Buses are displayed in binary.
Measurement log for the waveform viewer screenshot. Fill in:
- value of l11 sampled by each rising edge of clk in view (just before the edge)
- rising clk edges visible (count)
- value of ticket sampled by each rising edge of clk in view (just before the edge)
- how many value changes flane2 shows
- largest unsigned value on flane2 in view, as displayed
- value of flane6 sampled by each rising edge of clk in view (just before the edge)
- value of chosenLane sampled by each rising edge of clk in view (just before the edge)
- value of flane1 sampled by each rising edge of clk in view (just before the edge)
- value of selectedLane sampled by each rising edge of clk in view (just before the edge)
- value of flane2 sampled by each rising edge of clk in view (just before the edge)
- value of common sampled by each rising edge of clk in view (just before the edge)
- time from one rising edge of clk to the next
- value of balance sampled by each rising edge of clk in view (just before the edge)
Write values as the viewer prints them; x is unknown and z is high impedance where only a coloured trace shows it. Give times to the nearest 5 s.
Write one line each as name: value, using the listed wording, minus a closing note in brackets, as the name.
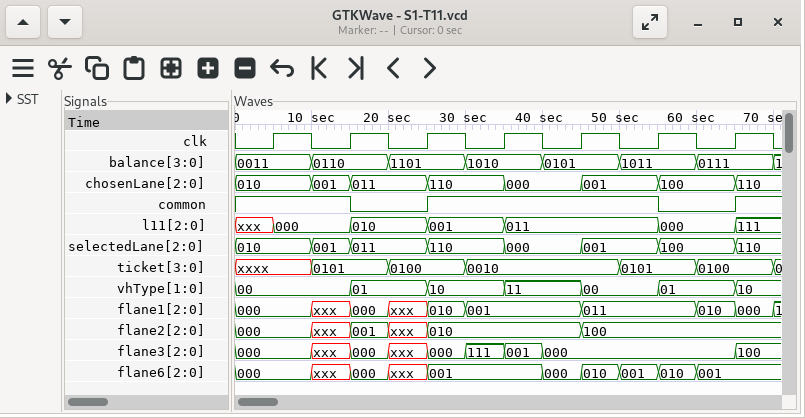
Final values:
value of l11 sampled by each rising edge of clk in view: xxx, 000, 010, 001, 011, 011, 000
rising clk edges visible: 7
value of ticket sampled by each rising edge of clk in view: xxxx, 0101, 0100, 0010, 0010, 0101, 0100
how many value changes flane2 shows: 5
largest unsigned value on flane2 in view, as displayed: 100
value of flane6 sampled by each rising edge of clk in view: 000, xxx, xxx, 001, 000, 001, 001
value of chosenLane sampled by each rising edge of clk in view: 010, 001, 011, 110, 000, 001, 100
value of flane1 sampled by each rising edge of clk in view: 000, xxx, xxx, 001, 001, 011, 010
value of selectedLane sampled by each rising edge of clk in view: 010, 001, 011, 110, 000, 001, 100
value of flane2 sampled by each rising edge of clk in view: 000, xxx, xxx, 010, 010, 100, 100
value of common sampled by each rising edge of clk in view: 1 1 0 1 1 1 0
time from one rising edge of clk to the next: 10 s
value of balance sampled by each rising edge of clk in view: 0011, 0110, 1101, 1010, 0101, 1011, 0111
